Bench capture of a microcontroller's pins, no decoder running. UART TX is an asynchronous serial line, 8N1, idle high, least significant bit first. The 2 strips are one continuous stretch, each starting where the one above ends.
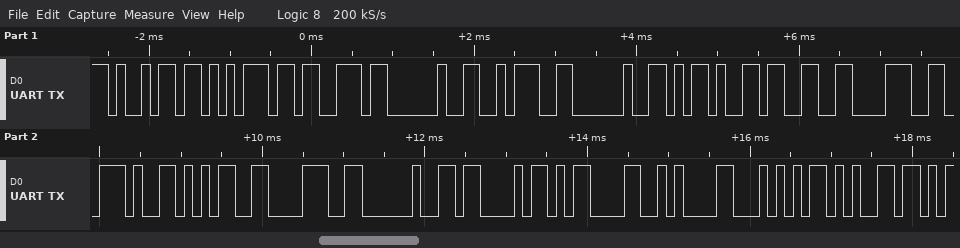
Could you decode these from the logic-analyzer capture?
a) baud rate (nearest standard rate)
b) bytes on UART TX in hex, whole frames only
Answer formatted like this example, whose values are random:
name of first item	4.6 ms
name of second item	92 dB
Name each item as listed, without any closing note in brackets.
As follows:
baud rate	9600 baud
bytes on UART TX in hex, whole frames only	0x69 0x75 0x73 0x20 0x3A 0x20 0x2D 0x33 0x38 0x2E 0x35 0x38 0x20 0x43 0x0D 0x0A 0x54 0x65
